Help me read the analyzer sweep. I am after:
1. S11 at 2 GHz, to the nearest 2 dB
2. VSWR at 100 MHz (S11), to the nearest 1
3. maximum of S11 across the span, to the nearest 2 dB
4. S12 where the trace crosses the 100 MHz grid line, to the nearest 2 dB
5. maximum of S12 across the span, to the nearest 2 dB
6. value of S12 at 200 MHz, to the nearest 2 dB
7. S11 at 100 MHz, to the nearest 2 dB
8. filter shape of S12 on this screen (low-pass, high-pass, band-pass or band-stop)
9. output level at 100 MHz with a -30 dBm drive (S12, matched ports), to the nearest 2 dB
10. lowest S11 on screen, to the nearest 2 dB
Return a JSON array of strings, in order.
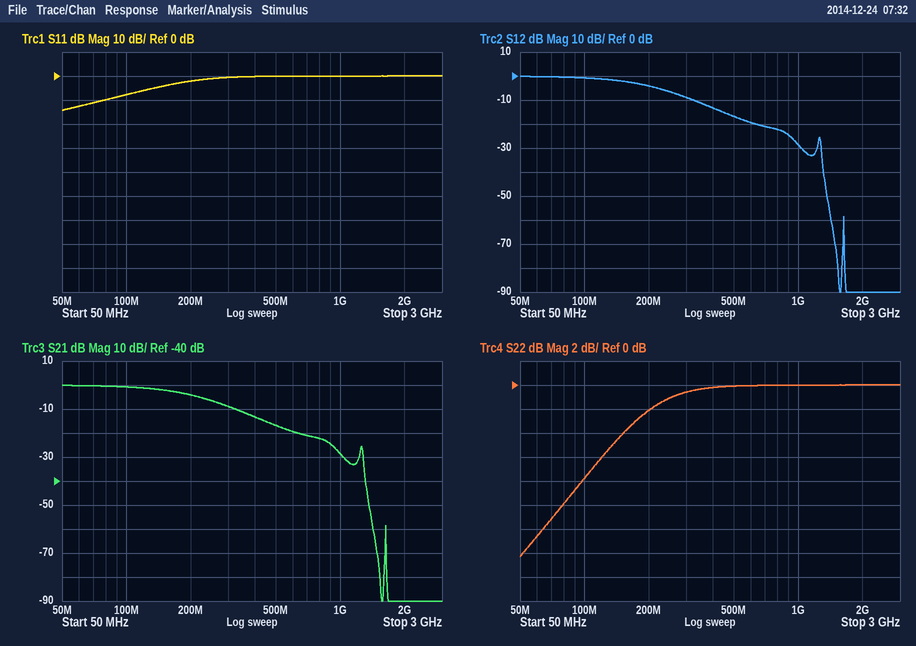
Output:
["0 dB", "2", "0 dB", "0 dB", "0 dB", "-4 dB", "-8 dB", "low-pass", "-30 dBm", "-14 dB"]
